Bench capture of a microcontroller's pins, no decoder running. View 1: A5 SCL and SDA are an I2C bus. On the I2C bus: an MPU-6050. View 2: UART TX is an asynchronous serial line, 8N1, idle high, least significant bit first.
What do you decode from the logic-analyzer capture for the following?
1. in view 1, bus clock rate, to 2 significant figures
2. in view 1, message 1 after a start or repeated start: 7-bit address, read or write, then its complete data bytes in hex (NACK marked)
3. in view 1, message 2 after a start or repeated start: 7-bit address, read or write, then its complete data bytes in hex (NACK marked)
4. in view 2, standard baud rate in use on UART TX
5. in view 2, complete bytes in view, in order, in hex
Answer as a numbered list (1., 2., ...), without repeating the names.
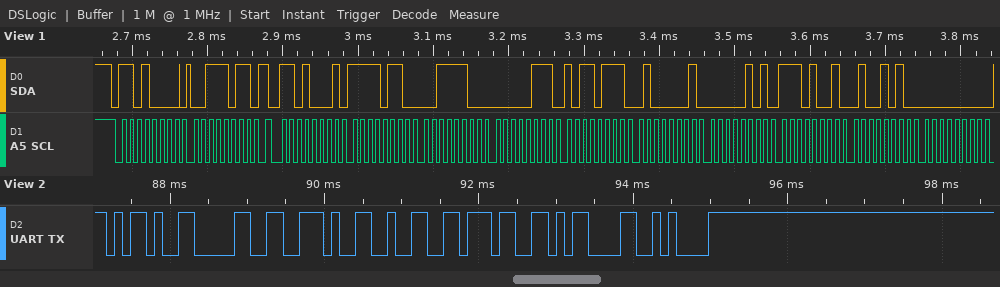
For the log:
1. 100 kHz
2. 0x68 write: 3B
3. 0x68 read: F6 3C 07 B7 41 05 E9 4A 00
4. 9600 baud
5. 2D 30 2E 32 37 0D 0A
